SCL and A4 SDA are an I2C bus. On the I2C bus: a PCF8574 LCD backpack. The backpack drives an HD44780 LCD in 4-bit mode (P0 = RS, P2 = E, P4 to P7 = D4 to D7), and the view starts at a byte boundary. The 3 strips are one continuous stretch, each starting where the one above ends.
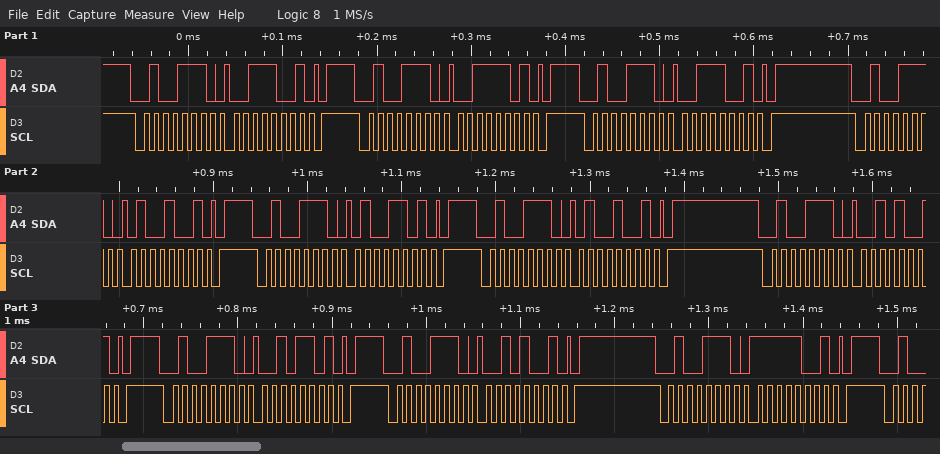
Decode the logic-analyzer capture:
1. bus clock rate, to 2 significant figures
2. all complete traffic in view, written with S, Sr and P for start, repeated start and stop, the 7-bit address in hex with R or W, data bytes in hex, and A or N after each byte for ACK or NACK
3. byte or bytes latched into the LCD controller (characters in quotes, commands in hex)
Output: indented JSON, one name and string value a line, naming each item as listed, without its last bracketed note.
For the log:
{
  "bus clock rate, to 2 significant figures": "100 kHz",
  "all complete traffic in view, written with S, Sr and P for start, repeated start and stop, the 7-bit address in hex with R or W, data bytes in hex, and A or N after each byte for ACK or NACK": "S 27W A 39 A P S 27W A 3D A P S 27W A 39 A P S 27W A 49 A P S 27W A 4D A P S 27W A 49 A P S 27W A 29 A P S 27W A 2D A P S 27W A 29 A P S 27W A F9 A P",
  "byte or bytes latched into the LCD controller": "'4'"
}
